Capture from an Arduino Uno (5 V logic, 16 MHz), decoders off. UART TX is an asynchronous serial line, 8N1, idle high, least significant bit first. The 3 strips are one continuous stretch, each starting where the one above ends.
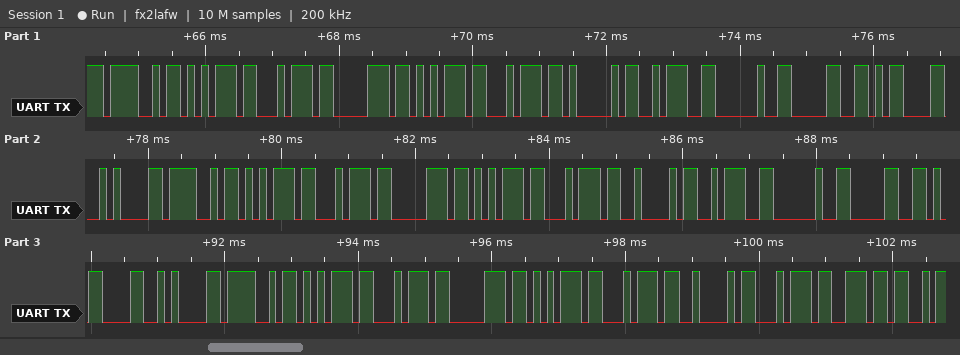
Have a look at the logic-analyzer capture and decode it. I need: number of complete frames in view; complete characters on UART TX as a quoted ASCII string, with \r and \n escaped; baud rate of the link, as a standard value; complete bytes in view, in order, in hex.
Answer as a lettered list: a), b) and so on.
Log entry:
a) 33
b) "OutputA: 0\r\nOutputB: 0\r\nOutputBtn"
c) 9600 baud
d) 0x4F 0x75 0x74 0x70 0x75 0x74 0x41 0x3A 0x20 0x30 0x0D 0x0A 0x4F 0x75 0x74 0x70 0x75 0x74 0x42 0x3A 0x20 0x30 0x0D 0x0A 0x4F 0x75 0x74 0x70 0x75 0x74 0x42 0x74 0x6E
